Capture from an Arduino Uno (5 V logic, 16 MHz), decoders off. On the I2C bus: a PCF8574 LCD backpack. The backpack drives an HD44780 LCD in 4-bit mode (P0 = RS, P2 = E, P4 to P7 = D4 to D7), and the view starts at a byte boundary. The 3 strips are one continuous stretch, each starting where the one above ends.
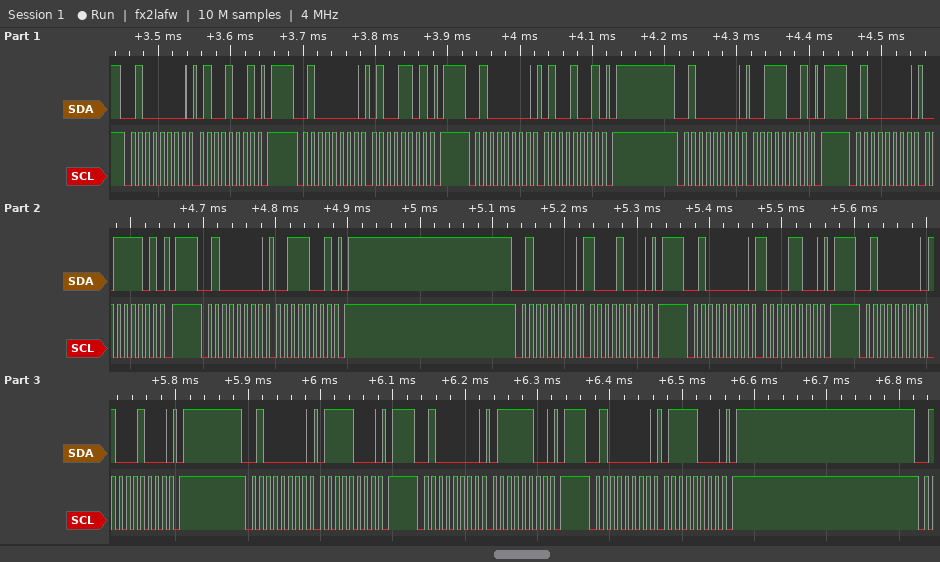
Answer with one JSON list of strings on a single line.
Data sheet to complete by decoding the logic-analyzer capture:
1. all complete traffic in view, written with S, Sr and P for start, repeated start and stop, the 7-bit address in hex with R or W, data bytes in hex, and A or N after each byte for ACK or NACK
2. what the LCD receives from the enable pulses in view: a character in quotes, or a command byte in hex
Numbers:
["S 20W A 49 A P S 20W A 4D A P S 20W A 49 A P S 20W A 39 A P S 20W A 3D A P S 20W A 39 A P S 20W A 88 A P S 20W A 8C A P S 20W A 88 A P S 20W A 78 A P S 20W A 7C A P S 20W A 78 A P", "'C' 0x87"]
